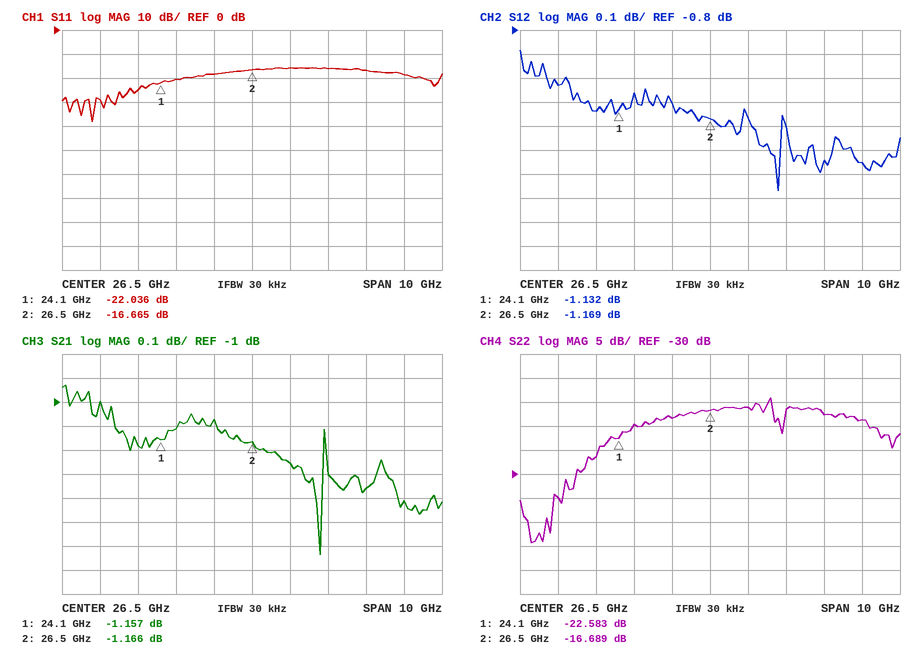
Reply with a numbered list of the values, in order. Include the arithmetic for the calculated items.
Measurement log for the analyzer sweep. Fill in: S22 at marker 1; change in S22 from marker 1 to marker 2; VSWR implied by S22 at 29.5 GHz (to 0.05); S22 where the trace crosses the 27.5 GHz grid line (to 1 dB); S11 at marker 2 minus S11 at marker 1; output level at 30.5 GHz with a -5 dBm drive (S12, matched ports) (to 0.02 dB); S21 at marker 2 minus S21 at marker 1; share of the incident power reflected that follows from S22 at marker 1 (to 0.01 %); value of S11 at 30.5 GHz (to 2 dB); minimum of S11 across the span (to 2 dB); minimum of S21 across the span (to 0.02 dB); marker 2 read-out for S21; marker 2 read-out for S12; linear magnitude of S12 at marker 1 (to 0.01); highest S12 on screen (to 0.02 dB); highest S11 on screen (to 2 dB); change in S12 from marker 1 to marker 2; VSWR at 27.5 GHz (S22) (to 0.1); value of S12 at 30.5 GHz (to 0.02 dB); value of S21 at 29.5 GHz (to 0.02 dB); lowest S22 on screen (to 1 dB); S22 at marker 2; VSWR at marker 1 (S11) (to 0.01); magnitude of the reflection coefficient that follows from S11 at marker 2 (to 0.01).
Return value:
1. -22.583 dB
2. -16.689 − (-22.583) = 5.894 dB
3. |Γ| = 10^(-18/20) = 0.1259; VSWR = (1 + 0.1259)/(1 − 0.1259) ≈ 1.29, so 1.30 to the nearest 0.05
4. -16 dB
5. -16.665 − (-22.036) = 5.371 dB
6. -5 dBm + (-1.36 dB) = -6.36 dBm
7. -1.166 − (-1.157) = -0.009 dB
8. 10^(-22.583/10) ≈ 0.55 %
9. -18 dB
10. -38 dB
11. -1.64 dB
12. -1.166 dB
13. -1.169 dB
14. 10^(-1.132/20) ≈ 0.88
15. -0.88 dB
16. -16 dB
17. -1.169 − (-1.132) = -0.037 dB
18. |Γ| = 10^(-16/20) = 0.1585; VSWR = (1 + 0.1585)/(1 − 0.1585) ≈ 1.4
19. -1.36 dB
20. -1.36 dB
21. -44 dB
22. -16.689 dB
23. (1 + 0.0791)/(1 − 0.0791) ≈ 1.17
24. 10^(-16.665/20) ≈ 0.15
